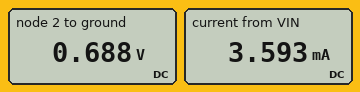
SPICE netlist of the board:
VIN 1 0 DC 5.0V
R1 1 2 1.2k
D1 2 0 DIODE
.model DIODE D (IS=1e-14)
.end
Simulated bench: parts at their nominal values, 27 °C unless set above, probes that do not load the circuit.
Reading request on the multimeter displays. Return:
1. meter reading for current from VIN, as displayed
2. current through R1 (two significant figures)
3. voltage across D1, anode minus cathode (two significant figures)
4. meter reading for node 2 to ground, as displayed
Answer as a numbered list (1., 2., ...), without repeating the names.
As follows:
1. 3.593 mA
2. 3.6 mA
3. 690 mV
4. 0.688 V
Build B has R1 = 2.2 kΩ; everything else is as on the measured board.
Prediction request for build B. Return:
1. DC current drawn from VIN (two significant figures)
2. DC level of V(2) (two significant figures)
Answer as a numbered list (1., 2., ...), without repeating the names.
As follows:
1. 2.0 mA
2. 670 mV
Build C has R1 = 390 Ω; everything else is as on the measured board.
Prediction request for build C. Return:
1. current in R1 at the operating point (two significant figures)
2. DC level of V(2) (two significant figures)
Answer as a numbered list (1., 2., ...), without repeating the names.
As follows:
1. 11 mA
2. 720 mV
